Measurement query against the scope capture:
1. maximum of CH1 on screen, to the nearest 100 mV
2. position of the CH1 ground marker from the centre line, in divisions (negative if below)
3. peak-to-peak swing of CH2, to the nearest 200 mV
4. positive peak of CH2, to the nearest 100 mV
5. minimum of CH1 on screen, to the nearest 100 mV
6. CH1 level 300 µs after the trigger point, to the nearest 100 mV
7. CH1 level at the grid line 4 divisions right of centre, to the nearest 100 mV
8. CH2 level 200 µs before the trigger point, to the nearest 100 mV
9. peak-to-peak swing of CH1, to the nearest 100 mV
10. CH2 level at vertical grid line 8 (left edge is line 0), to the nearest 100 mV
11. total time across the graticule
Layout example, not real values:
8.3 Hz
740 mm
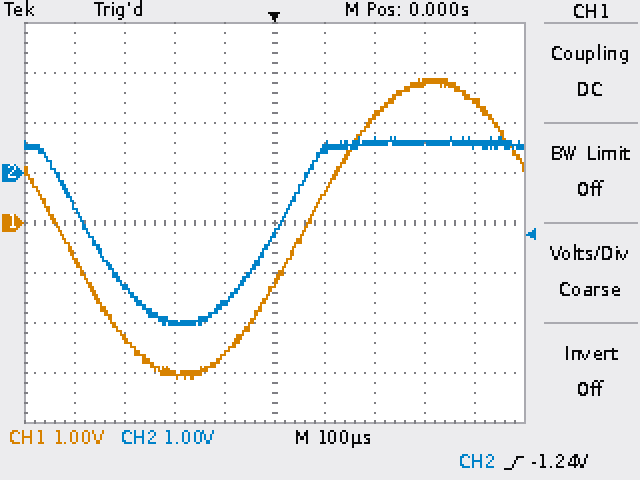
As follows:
2.9 V
0.0 div
3.8 V
700 mV
-3.1 V
2.8 V
2.4 V
-3.0 V
6.0 V
600 mV
1 ms
